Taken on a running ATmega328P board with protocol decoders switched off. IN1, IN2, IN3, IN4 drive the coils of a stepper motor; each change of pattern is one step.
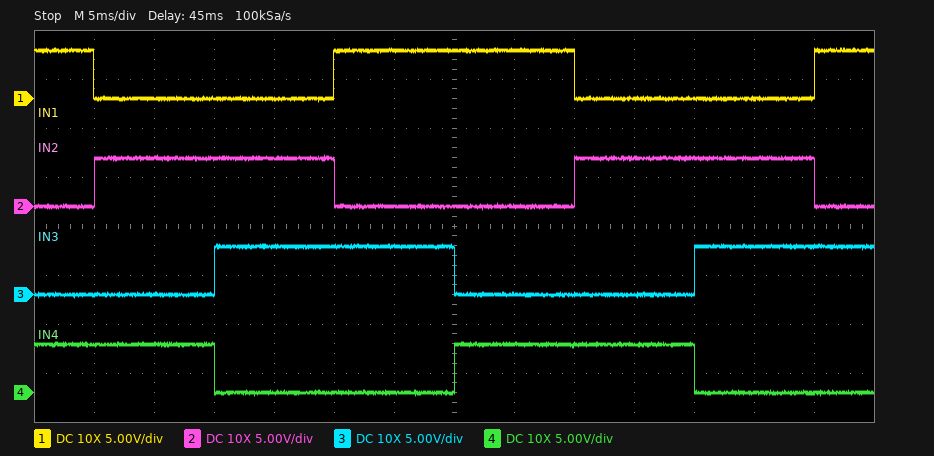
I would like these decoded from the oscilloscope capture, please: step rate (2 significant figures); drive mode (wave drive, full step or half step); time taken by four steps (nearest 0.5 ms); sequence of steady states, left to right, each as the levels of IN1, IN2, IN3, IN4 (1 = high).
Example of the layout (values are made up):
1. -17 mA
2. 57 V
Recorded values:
1. 100 steps/s
2. full step
3. 40.0 ms
4. 1001 0101 0110 1010 1001 0101 0110 1010
